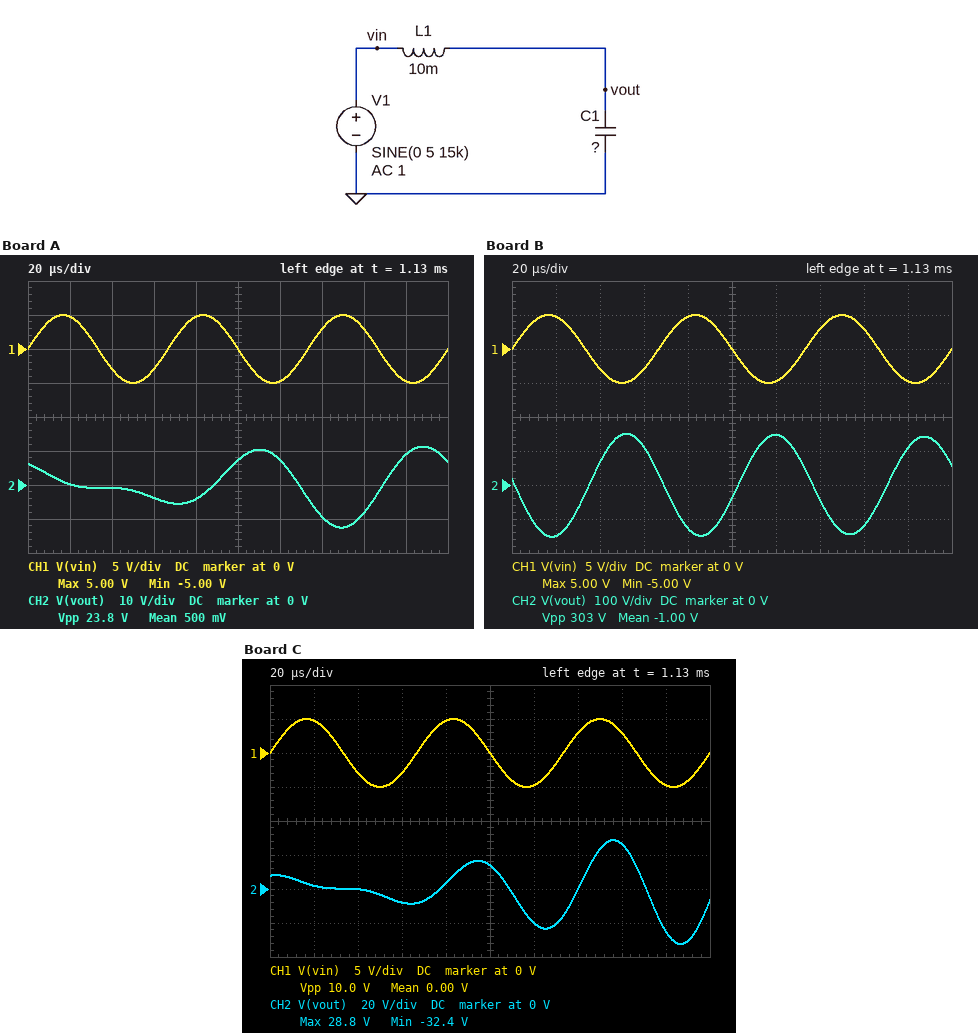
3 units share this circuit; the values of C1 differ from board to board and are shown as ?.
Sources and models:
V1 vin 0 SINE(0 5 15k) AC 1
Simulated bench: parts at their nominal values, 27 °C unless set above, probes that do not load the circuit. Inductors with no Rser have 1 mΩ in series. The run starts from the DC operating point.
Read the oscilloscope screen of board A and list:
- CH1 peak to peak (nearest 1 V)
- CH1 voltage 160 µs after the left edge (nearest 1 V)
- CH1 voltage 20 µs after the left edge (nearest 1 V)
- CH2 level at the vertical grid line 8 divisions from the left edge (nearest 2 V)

10 V
3 V
5 V
-8 V
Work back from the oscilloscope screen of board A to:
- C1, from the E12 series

22 nF
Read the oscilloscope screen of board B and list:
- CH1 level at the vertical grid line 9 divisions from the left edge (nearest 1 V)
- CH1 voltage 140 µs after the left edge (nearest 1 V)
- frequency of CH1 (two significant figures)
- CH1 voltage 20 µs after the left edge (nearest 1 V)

-5 V
3 V
15 kHz
5 V
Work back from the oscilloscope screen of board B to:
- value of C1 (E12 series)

12 nF
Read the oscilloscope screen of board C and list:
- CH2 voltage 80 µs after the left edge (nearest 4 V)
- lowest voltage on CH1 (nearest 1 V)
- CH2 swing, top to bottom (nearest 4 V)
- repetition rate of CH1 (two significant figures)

4 V
-5 V
60 V
15 kHz
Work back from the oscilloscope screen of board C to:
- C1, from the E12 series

8.2 nF
